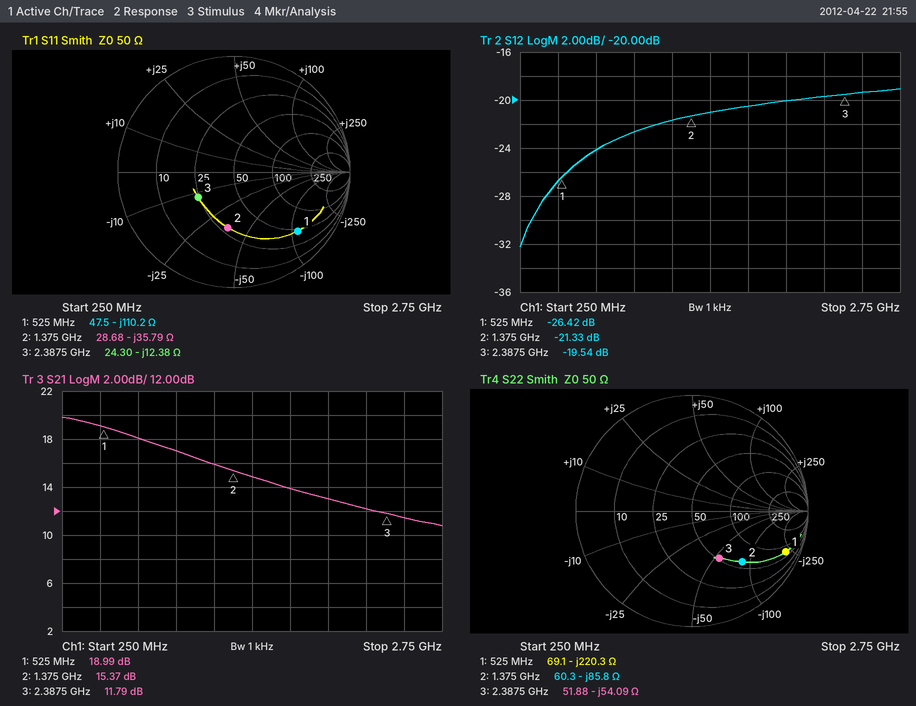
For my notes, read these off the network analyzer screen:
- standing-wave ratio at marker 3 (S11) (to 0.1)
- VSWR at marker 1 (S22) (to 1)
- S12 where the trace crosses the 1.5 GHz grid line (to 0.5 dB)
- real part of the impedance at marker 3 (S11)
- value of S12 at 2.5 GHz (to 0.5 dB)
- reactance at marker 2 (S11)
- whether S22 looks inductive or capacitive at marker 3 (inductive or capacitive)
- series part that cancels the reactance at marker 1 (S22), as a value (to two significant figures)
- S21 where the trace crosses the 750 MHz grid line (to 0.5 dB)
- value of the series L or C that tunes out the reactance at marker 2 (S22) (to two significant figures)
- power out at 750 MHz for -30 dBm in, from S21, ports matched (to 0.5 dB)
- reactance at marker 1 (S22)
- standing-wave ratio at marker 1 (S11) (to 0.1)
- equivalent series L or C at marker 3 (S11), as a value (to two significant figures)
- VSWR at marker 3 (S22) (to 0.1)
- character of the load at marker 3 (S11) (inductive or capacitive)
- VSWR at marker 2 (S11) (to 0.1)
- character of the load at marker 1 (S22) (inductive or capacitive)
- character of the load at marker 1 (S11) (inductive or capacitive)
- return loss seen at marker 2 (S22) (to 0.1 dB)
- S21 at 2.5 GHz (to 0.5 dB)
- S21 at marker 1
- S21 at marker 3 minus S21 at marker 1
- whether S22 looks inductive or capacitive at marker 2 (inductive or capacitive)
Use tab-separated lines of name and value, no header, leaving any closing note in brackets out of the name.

standing-wave ratio at marker 3 (S11)	2.2
VSWR at marker 1 (S22)	16
S12 where the trace crosses the 1.5 GHz grid line	-21.0 dB
real part of the impedance at marker 3	24.30 Ω
value of S12 at 2.5 GHz	-19.5 dB
reactance at marker 2	-35.79 Ω
whether S22 looks inductive or capacitive at marker 3	capacitive
series part that cancels the reactance at marker 1 (S22), as a value	67 nH
S21 where the trace crosses the 750 MHz grid line	18.0 dB
value of the series L or C that tunes out the reactance at marker 2 (S22)	9.9 nH
power out at 750 MHz for -30 dBm in, from S21, ports matched	-12.0 dBm
reactance at marker 1	-220.3 Ω
standing-wave ratio at marker 1 (S11)	7.0
equivalent series L or C at marker 3 (S11), as a value	5.4 pF
VSWR at marker 3 (S22)	2.8
character of the load at marker 3 (S11)	capacitive
VSWR at marker 2 (S11)	2.9
character of the load at marker 1 (S22)	capacitive
character of the load at marker 1 (S11)	capacitive
return loss seen at marker 2 (S22)	4.2 dB
S21 at 2.5 GHz	11.5 dB
S21 at marker 1	18.99 dB
S21 at marker 3 minus S21 at marker 1	-7.20 dB
whether S22 looks inductive or capacitive at marker 2	capacitive
